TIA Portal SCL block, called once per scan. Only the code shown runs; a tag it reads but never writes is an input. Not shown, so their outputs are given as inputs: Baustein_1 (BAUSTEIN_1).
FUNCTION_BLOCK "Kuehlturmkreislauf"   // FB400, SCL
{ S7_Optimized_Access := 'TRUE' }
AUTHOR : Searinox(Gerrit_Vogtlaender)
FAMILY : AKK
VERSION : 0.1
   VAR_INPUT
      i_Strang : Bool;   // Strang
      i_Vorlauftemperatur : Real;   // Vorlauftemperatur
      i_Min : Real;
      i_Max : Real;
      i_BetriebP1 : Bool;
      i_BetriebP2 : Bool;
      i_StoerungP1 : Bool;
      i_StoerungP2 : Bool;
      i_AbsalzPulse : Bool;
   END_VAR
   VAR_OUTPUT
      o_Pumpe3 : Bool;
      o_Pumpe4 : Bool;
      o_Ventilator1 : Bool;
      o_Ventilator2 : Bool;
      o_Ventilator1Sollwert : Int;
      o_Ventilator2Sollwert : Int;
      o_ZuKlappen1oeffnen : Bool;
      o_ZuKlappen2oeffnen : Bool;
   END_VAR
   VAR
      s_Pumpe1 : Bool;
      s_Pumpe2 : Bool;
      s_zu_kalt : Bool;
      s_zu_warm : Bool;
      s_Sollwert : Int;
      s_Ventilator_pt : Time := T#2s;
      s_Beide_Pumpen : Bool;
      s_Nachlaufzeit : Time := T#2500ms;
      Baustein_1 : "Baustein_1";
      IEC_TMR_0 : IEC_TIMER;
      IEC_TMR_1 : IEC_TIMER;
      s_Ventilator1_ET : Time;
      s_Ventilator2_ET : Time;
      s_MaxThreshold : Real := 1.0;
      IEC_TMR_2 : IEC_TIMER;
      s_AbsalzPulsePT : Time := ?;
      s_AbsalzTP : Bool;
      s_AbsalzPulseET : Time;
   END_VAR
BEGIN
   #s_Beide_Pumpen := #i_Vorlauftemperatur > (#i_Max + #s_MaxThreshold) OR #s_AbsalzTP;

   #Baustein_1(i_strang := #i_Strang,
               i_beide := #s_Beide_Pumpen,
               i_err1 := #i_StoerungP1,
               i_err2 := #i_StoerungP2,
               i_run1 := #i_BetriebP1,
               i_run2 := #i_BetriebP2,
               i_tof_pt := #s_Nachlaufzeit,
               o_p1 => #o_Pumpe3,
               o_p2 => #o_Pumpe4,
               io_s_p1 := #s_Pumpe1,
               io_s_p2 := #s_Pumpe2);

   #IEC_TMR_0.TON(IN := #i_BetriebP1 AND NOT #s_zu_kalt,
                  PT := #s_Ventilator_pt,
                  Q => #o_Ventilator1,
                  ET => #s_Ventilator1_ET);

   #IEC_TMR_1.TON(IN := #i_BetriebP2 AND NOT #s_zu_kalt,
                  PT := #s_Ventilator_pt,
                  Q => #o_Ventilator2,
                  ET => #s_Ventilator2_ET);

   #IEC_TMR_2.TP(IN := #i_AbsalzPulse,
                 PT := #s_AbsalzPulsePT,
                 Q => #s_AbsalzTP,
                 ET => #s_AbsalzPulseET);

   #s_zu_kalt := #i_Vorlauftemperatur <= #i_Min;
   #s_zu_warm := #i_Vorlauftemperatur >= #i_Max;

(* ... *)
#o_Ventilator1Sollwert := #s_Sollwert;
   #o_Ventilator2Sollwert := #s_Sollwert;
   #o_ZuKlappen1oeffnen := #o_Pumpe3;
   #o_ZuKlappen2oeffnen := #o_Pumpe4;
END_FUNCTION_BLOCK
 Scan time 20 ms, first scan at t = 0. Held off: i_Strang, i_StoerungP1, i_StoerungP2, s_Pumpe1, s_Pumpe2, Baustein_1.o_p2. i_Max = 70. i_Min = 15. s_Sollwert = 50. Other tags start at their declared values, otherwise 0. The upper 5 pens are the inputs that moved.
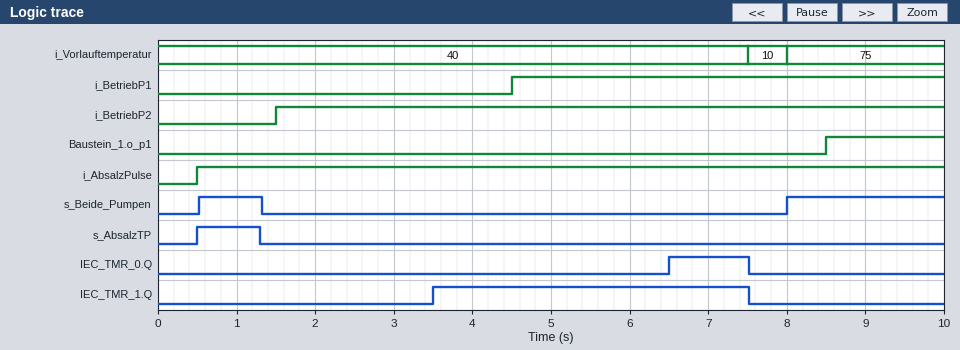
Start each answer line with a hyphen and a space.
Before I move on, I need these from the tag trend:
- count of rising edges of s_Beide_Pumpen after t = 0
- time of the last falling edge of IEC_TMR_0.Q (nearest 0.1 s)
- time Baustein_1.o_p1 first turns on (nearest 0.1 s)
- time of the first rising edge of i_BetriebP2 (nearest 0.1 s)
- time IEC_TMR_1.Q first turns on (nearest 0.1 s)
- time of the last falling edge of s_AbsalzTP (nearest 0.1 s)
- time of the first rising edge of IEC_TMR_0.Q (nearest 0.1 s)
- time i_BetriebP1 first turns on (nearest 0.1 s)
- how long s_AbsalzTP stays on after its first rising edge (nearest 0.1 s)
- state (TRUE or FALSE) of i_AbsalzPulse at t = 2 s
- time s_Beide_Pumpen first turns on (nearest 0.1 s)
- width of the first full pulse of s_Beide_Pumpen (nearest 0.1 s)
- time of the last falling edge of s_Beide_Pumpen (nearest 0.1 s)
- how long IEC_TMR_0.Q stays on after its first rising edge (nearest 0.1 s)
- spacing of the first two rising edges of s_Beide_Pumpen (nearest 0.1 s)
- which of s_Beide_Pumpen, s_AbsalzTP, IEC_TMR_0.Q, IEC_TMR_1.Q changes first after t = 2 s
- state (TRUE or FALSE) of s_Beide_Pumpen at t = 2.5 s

- 2
- 7.5 s
- 8.5 s
- 1.5 s
- 3.5 s
- 1.3 s
- 6.5 s
- 4.5 s
- 0.8 s
- TRUE
- 0.5 s
- 0.8 s
- 1.3 s
- 1.0 s
- 7.5 s
- IEC_TMR_1.Q
- FALSE
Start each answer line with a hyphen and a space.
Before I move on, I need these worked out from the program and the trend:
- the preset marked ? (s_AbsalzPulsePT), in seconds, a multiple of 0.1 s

- 0.8 s
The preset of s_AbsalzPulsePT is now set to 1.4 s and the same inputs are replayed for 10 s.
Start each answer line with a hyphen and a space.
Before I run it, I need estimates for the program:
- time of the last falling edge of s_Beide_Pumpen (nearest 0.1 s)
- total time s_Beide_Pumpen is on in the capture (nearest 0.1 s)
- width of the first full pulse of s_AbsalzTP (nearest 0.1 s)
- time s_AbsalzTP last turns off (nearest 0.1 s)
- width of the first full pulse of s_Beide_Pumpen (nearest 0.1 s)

- 1.9 s
- 3.4 s
- 1.4 s
- 1.9 s
- 1.4 s
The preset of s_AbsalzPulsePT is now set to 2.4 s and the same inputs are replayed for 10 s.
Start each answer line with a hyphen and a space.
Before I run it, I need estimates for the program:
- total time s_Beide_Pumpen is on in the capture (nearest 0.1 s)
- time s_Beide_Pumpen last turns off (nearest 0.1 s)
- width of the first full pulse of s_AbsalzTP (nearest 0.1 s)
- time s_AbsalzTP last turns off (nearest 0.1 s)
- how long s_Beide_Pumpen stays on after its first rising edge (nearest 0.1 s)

- 4.4 s
- 2.9 s
- 2.4 s
- 2.9 s
- 2.4 s
